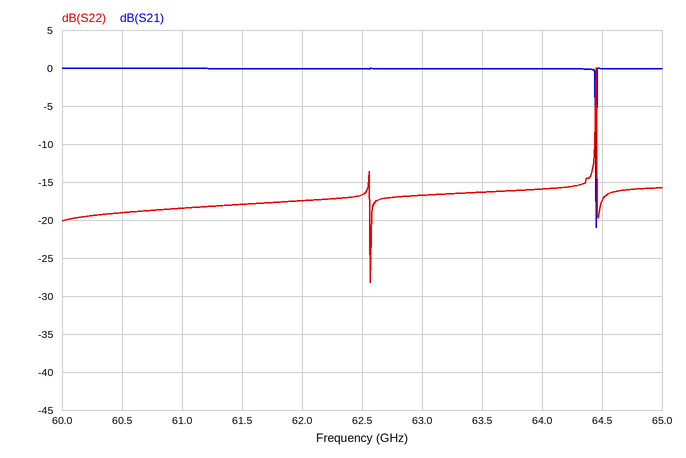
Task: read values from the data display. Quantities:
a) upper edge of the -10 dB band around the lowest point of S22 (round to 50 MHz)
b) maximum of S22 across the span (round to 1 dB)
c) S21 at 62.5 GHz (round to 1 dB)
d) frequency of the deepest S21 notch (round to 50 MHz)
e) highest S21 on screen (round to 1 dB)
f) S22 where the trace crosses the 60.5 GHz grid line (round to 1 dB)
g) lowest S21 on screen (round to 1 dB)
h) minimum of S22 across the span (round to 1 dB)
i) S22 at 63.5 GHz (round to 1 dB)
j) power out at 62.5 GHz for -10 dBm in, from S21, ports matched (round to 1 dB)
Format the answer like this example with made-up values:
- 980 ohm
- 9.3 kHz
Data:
- 64.45 GHz
- 0 dB
- 0 dB
- 64.45 GHz
- 0 dB
- -19 dB
- -21 dB
- -28 dB
- -16 dB
- -10 dBm
